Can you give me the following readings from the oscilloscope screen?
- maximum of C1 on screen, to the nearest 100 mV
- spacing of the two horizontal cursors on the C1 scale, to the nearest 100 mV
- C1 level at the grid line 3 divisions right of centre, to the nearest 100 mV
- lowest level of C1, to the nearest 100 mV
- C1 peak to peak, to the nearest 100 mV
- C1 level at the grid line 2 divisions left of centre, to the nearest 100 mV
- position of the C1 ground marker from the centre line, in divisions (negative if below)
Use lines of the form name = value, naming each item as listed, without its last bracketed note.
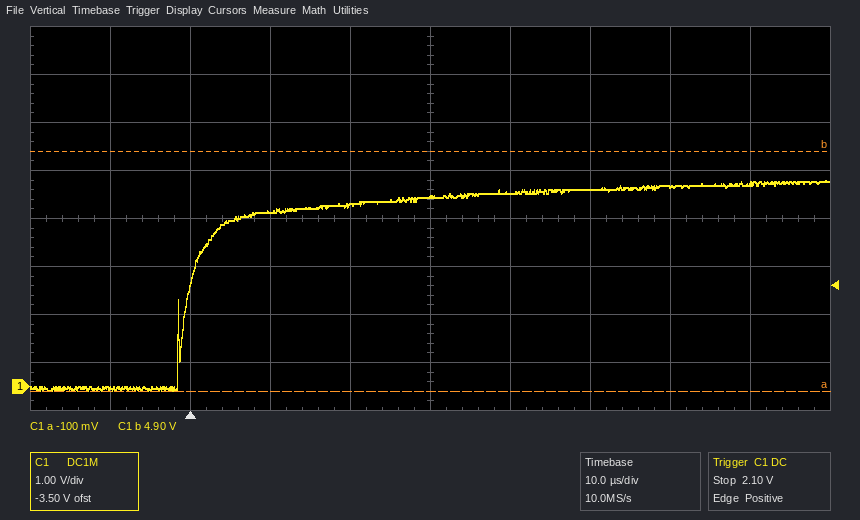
maximum of C1 on screen, to the nearest 100 mV = 4.3 V
spacing of the two horizontal cursors on the C1 scale, to the nearest 100 mV = 5.0 V
C1 level at the grid line 3 divisions right of centre, to the nearest 100 mV = 4.2 V
lowest level of C1, to the nearest 100 mV = -100 mV
C1 peak to peak, to the nearest 100 mV = 4.4 V
C1 level at the grid line 2 divisions left of centre, to the nearest 100 mV = 3.6 V
position of the C1 ground marker from the centre line, in divisions = -3.5 div
